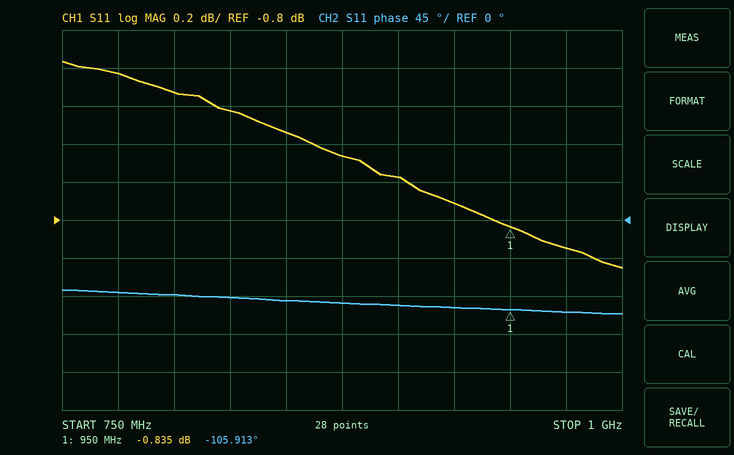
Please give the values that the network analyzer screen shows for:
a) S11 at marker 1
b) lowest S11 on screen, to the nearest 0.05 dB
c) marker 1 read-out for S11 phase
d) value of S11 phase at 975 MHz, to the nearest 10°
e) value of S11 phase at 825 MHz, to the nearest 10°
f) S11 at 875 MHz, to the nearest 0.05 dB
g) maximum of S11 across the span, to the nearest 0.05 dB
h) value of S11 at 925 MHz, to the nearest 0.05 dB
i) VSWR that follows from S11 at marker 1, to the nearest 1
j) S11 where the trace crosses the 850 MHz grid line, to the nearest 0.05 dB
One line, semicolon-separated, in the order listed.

-0.835 dB; -1.05 dB; -105.913°; -110°; -90°; -0.45 dB; 0.05 dB; -0.70 dB; 21; -0.35 dB
